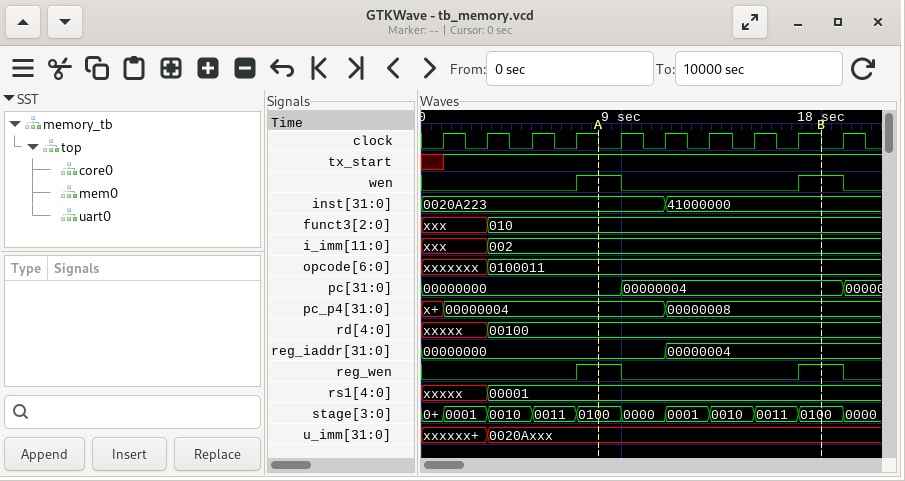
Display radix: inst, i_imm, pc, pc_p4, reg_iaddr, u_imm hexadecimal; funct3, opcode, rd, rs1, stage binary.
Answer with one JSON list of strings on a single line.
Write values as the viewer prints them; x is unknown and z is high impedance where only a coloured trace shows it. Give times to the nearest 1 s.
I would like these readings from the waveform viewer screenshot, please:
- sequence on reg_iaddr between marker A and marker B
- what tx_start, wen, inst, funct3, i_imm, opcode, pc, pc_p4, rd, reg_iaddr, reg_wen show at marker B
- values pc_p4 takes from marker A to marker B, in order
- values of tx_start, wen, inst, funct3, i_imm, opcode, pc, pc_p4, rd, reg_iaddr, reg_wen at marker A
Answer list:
["00000000, 00000004", "tx_start=1, wen=1, inst=41000000, funct3=010, i_imm=002, opcode=0100011, pc=00000004, pc_p4=00000008, rd=00100, reg_iaddr=00000004, reg_wen=1", "00000004, 00000008", "tx_start=1, wen=1, inst=0020A223, funct3=010, i_imm=002, opcode=0100011, pc=00000000, pc_p4=00000004, rd=00100, reg_iaddr=00000000, reg_wen=1"]
